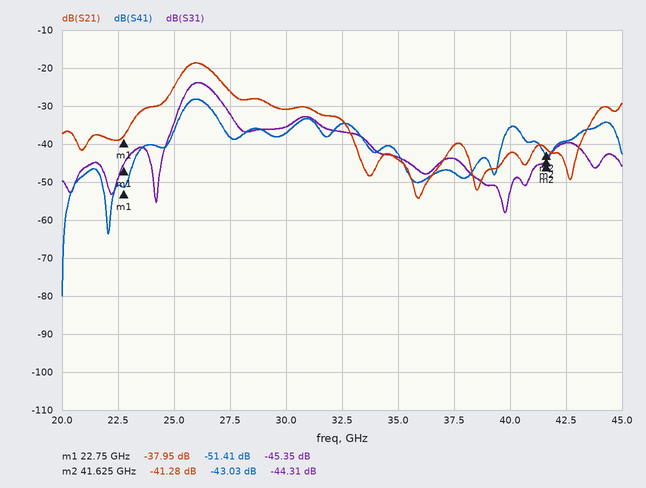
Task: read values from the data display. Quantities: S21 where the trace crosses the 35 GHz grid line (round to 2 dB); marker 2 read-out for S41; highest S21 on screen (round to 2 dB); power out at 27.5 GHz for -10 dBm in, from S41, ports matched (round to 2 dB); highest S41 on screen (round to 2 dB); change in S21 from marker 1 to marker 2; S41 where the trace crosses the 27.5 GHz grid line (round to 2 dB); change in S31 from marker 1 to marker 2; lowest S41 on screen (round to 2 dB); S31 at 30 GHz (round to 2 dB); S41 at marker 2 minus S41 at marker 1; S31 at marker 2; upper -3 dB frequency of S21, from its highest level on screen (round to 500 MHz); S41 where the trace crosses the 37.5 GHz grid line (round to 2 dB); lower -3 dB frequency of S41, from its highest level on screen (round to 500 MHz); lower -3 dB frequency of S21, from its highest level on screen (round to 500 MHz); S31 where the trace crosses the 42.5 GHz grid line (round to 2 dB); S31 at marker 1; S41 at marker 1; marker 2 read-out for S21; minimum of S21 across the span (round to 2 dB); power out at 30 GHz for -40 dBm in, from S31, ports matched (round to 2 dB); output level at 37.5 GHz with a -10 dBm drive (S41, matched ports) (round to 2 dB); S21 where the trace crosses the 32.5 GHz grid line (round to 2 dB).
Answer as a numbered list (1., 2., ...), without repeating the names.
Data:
1. -44 dB
2. -43.03 dB
3. -18 dB
4. -48 dBm
5. -28 dB
6. -3.33 dB
7. -38 dB
8. 1.04 dB
9. -80 dB
10. -36 dB
11. 8.38 dB
12. -44.31 dB
13. 27.0 GHz
14. -48 dB
15. 25.5 GHz
16. 25.5 GHz
17. -40 dB
18. -45.35 dB
19. -51.41 dB
20. -41.28 dB
21. -54 dB
22. -76 dBm
23. -58 dBm
24. -34 dB
